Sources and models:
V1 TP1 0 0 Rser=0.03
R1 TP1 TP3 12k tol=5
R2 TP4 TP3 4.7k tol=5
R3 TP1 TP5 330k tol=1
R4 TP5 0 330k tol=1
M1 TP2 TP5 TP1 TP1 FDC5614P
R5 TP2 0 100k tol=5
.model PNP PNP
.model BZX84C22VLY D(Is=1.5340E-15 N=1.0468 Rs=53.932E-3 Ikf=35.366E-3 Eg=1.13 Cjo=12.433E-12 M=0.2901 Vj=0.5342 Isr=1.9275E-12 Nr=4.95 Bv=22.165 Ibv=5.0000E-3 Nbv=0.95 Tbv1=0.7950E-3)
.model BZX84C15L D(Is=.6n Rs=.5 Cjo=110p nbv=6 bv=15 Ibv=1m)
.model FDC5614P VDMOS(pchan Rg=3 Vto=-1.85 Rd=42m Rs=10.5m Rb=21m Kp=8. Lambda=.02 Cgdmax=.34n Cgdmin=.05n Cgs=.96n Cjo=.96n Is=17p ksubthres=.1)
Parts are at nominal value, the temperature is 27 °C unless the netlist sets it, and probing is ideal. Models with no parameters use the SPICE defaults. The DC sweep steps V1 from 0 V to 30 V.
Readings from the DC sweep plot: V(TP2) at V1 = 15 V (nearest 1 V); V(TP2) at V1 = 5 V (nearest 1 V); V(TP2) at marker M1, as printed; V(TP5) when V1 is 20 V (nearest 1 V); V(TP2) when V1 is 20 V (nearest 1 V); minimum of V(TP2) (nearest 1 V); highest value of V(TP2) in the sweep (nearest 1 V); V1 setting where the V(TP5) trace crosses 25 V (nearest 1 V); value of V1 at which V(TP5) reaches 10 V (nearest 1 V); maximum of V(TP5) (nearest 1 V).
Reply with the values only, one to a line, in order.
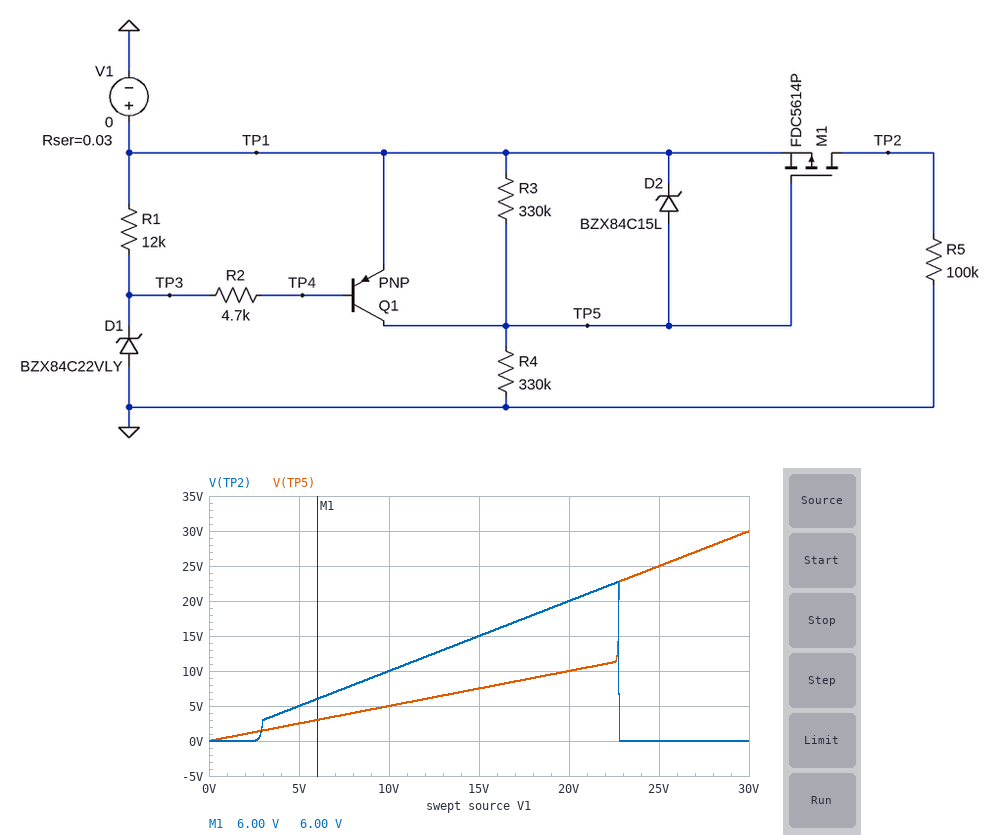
15 V
5 V
6.00 V
10 V
20 V
0 V
23 V
25 V
20 V
30 V
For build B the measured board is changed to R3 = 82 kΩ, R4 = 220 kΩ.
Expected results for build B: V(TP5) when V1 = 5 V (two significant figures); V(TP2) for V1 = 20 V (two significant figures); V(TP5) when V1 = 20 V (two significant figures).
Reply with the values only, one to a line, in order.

3.6 V
20 V
15 V
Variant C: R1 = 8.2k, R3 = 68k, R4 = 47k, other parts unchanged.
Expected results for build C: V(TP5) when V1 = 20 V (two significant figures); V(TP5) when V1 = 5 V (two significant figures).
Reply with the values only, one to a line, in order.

8.2 V
2.0 V
